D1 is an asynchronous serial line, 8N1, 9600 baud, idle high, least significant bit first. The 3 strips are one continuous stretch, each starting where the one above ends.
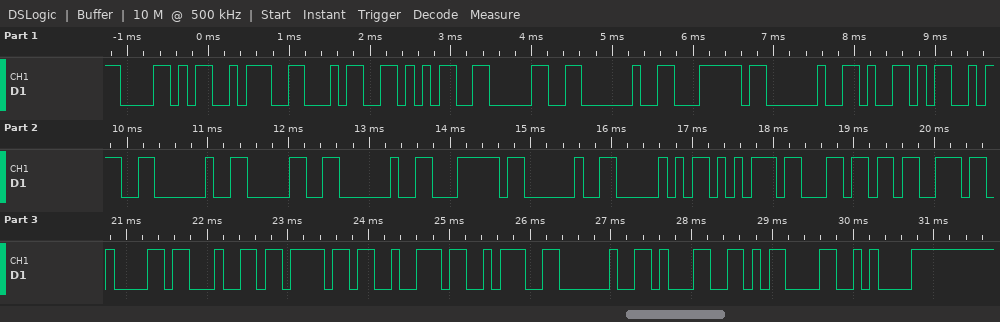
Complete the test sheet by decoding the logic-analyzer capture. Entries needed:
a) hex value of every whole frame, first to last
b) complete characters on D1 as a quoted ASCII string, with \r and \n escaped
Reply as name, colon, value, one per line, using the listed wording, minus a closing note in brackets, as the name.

hex value of every whole frame, first to last: 58 3A 34 35 30 20 7C 20 59 3A 20 30 20 7C 20 50 75 6C 73 61 64 6F 72 3A 20 31 0D 0A
complete characters on D1 as a quoted ASCII string, with \r and \n escaped: "X:450 | Y: 0 | Pulsador: 1\r\n"
